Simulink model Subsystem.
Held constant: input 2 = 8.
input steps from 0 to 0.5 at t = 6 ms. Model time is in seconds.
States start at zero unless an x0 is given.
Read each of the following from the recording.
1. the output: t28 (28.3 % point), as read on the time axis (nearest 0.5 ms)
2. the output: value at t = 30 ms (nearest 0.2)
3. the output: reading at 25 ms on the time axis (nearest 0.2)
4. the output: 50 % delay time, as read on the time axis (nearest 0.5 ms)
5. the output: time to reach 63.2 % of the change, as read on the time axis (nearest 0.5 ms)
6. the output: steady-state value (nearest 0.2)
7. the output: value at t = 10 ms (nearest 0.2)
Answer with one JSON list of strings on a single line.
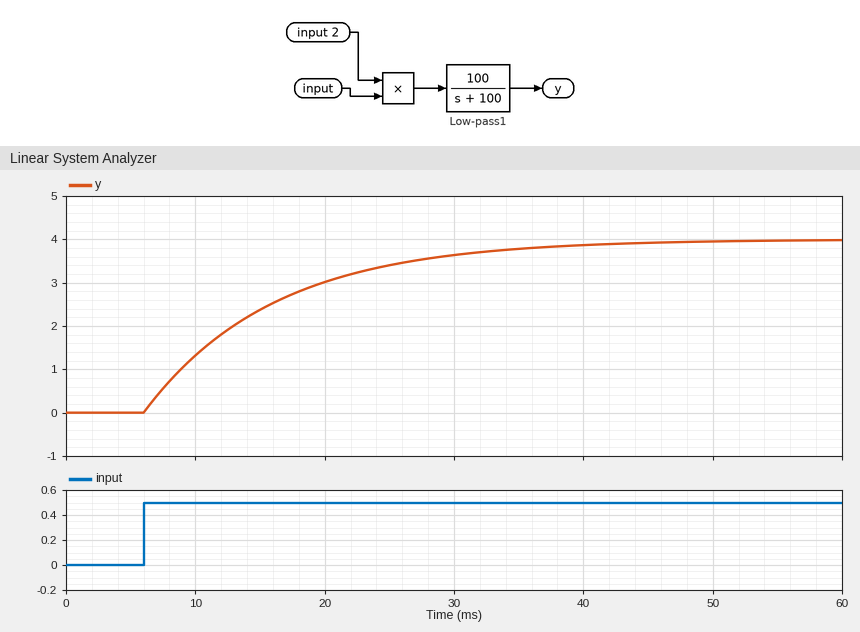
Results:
["9.5 ms", "3.6", "3.4", "13.0 ms", "16.0 ms", "4.0", "1.4"]
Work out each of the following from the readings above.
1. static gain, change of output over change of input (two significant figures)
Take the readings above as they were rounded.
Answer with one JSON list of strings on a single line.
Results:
["8.0"]
